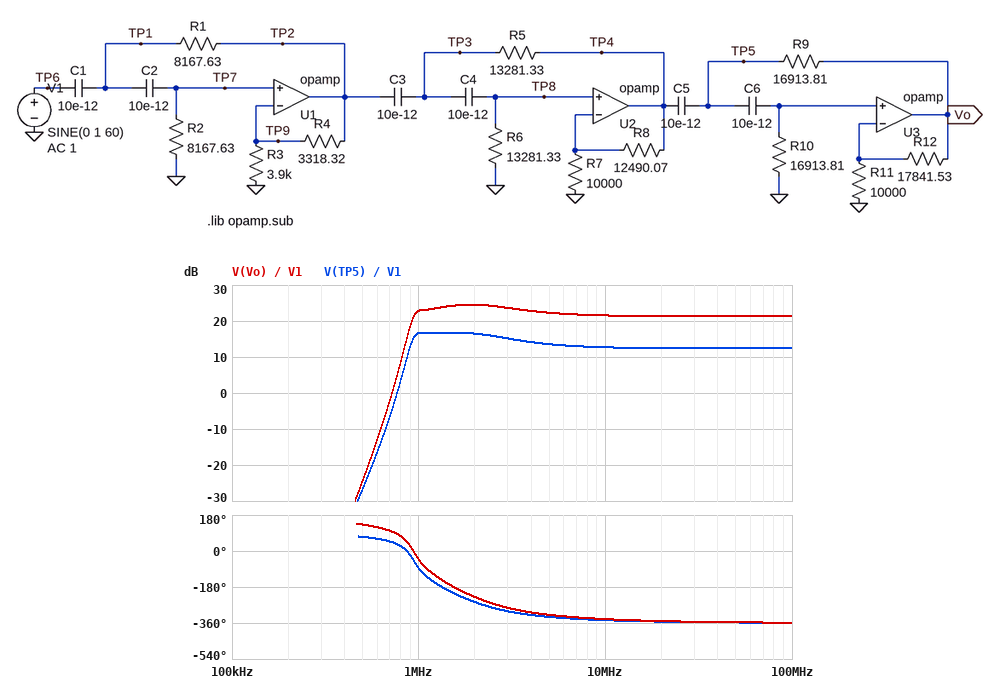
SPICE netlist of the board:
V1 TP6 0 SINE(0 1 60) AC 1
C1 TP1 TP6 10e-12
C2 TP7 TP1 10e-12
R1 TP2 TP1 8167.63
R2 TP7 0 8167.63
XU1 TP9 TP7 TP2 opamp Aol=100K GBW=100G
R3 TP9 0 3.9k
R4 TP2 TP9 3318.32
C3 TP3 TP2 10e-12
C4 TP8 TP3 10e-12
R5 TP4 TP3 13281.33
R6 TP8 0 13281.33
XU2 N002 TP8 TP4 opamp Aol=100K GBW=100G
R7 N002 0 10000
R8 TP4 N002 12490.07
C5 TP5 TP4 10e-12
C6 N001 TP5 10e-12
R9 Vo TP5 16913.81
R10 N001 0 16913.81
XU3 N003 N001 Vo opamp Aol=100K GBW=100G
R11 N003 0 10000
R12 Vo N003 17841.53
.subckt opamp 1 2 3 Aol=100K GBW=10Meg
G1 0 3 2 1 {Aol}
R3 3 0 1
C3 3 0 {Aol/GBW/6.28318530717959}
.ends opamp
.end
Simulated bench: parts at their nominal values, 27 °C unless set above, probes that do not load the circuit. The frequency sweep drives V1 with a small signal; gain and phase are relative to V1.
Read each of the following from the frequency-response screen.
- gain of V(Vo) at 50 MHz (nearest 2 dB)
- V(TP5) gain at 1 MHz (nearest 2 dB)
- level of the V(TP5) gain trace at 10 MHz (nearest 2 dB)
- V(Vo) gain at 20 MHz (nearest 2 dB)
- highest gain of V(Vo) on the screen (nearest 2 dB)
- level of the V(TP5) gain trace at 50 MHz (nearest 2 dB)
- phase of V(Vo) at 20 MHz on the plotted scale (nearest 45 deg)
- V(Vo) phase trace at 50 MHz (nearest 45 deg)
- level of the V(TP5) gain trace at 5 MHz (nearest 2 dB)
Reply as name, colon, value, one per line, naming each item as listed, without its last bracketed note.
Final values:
gain of V(Vo) at 50 MHz: 22 dB
V(TP5) gain at 1 MHz: 16 dB
level of the V(TP5) gain trace at 10 MHz: 12 dB
V(Vo) gain at 20 MHz: 22 dB
highest gain of V(Vo) on the screen: 24 dB
level of the V(TP5) gain trace at 50 MHz: 12 dB
phase of V(Vo) at 20 MHz on the plotted scale: -360 deg
V(Vo) phase trace at 50 MHz: -360 deg
level of the V(TP5) gain trace at 5 MHz: 14 dB
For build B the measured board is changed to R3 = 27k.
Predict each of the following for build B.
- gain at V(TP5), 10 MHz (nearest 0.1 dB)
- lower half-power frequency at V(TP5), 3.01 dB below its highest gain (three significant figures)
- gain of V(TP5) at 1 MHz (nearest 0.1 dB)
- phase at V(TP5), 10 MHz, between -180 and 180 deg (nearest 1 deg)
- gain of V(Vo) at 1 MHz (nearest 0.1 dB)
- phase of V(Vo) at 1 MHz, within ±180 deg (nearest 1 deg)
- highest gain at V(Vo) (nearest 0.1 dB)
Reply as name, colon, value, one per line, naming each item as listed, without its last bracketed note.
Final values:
gain at V(TP5), 10 MHz: 8.0 dB
lower half-power frequency at V(TP5), 3.01 dB below its highest gain: 907 kHz
gain of V(TP5) at 1 MHz: 10.2 dB
phase at V(TP5), 10 MHz, between -180 and 180 deg: 22 deg
gain of V(Vo) at 1 MHz: 16.3 dB
phase of V(Vo) at 1 MHz, within ±180 deg: -56 deg
highest gain at V(Vo): 16.9 dB
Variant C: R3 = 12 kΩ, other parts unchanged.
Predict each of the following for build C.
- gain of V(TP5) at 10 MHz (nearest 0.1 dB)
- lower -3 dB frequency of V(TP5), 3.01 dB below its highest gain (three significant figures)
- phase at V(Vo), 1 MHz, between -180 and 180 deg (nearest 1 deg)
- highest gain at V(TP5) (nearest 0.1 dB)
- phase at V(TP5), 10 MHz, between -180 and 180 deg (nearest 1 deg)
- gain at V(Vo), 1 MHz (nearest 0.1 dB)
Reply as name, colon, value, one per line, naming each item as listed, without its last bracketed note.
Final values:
gain of V(TP5) at 10 MHz: 9.2 dB
lower -3 dB frequency of V(TP5), 3.01 dB below its highest gain: 908 kHz
phase at V(Vo), 1 MHz, between -180 and 180 deg: -54 deg
highest gain at V(TP5): 11.8 dB
phase at V(TP5), 10 MHz, between -180 and 180 deg: 20 deg
gain at V(Vo), 1 MHz: 17.9 dB
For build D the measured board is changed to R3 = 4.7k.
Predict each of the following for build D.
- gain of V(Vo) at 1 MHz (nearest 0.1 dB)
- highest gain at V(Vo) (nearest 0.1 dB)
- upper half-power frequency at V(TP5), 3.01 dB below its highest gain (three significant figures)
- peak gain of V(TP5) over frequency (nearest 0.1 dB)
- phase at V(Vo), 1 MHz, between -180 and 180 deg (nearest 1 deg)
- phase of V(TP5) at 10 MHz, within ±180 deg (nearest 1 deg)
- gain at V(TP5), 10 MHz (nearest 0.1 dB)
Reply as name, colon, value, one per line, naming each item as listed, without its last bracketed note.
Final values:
gain of V(Vo) at 1 MHz: 21.7 dB
highest gain at V(Vo): 22.8 dB
upper half-power frequency at V(TP5), 3.01 dB below its highest gain: 5.05 MHz
peak gain of V(TP5) over frequency: 15.6 dB
phase at V(Vo), 1 MHz, between -180 and 180 deg: -46 deg
phase of V(TP5) at 10 MHz, within ±180 deg: 16 deg
gain at V(TP5), 10 MHz: 11.9 dB
